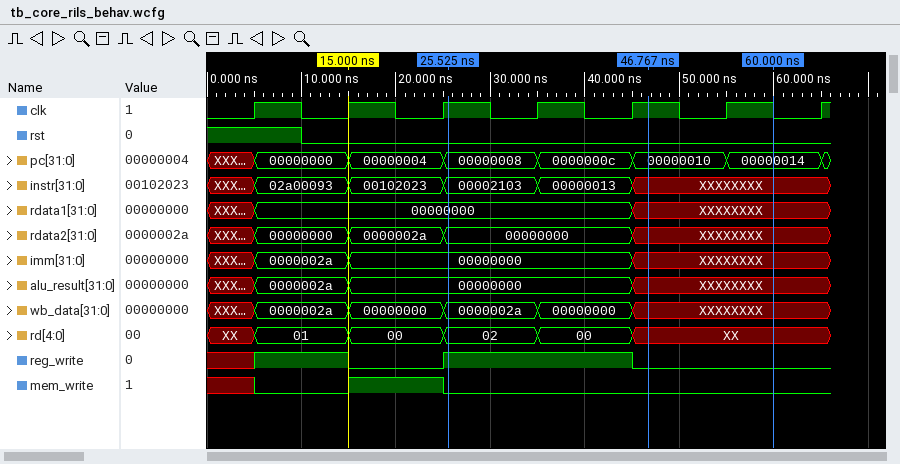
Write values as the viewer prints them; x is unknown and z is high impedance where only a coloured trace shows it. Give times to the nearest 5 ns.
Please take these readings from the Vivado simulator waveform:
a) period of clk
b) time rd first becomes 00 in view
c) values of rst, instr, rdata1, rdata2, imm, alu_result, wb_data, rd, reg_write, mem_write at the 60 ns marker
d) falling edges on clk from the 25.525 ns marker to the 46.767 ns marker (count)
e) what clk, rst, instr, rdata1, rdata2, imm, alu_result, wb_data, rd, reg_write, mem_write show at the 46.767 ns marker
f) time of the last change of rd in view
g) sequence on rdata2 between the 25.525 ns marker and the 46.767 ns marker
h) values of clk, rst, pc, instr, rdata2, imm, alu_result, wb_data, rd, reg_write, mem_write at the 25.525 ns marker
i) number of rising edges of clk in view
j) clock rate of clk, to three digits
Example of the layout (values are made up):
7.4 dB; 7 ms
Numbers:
10 ns; 15 ns; rst=0, instr=XXXXXXXX, rdata1=XXXXXXXX, rdata2=XXXXXXXX, imm=XXXXXXXX, alu_result=XXXXXXXX, wb_data=XXXXXXXX, rd=XX, reg_write=0, mem_write=0; 2; clk=1, rst=0, instr=XXXXXXXX, rdata1=XXXXXXXX, rdata2=XXXXXXXX, imm=XXXXXXXX, alu_result=XXXXXXXX, wb_data=XXXXXXXX, rd=XX, reg_write=0, mem_write=0; 45 ns; 00000000, XXXXXXXX; clk=1, rst=0, pc=00000008, instr=00002103, rdata2=00000000, imm=00000000, alu_result=00000000, wb_data=0000002a, rd=02, reg_write=1, mem_write=0; 7; 100 MHz
